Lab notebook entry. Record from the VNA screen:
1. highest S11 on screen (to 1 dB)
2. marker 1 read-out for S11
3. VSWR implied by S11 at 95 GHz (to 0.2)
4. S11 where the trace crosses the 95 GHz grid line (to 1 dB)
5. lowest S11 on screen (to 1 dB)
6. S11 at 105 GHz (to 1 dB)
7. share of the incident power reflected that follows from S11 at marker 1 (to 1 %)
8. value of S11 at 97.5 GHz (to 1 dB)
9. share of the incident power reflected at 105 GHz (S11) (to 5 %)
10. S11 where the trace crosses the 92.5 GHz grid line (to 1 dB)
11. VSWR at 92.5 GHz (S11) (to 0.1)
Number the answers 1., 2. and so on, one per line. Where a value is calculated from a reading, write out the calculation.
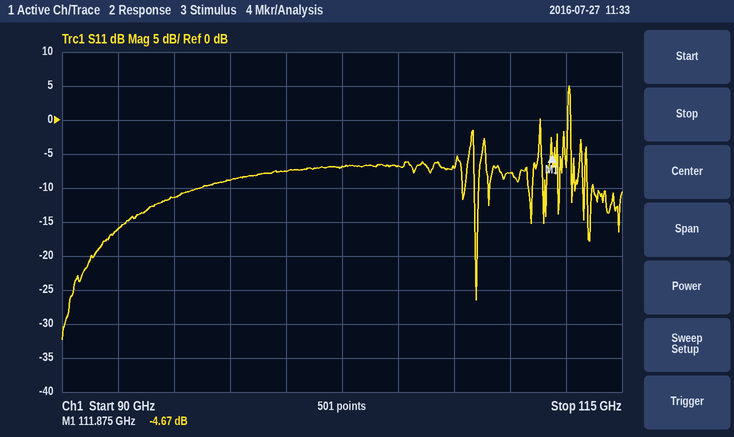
1. 5 dB
2. -4.67 dB
3. |Γ| = 10^(-11/20) = 0.2818; VSWR = (1 + 0.2818)/(1 − 0.2818) ≈ 1.8
4. -11 dB
5. -32 dB
6. -7 dB
7. 10^(-4.67/10) ≈ 34 %
8. -9 dB
9. 10^(-7/10) ≈ 20 %
10. -16 dB
11. |Γ| = 10^(-16/20) = 0.1585; VSWR = (1 + 0.1585)/(1 − 0.1585) ≈ 1.4
